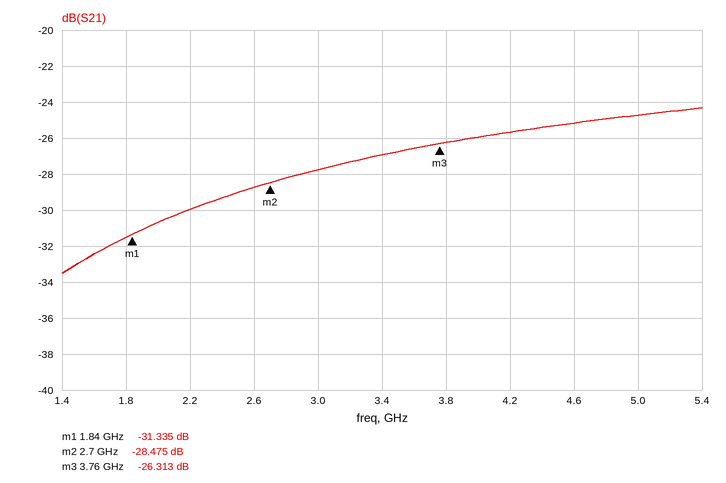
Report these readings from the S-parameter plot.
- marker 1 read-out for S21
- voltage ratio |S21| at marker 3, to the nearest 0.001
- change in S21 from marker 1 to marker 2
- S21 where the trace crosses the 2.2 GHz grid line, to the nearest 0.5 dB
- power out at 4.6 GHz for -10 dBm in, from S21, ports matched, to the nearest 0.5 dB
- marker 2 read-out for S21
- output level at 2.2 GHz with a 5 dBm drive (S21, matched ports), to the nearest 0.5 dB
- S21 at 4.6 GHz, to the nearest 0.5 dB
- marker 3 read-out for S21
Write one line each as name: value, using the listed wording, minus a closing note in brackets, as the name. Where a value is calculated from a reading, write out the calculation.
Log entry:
marker 1 read-out for S21: -31.335 dB
voltage ratio |S21| at marker 3, to the nearest 0.001: 10^(-26.313/20) ≈ 0.048
change in S21 from marker 1 to marker 2: -28.475 − (-31.335) = 2.860 dB
S21 where the trace crosses the 2.2 GHz grid line, to the nearest 0.5 dB: -30.0 dB
power out at 4.6 GHz for -10 dBm in, from S21, ports matched, to the nearest 0.5 dB: -10 dBm + (-25.0 dB) = -35.0 dBm
marker 2 read-out for S21: -28.475 dB
output level at 2.2 GHz with a 5 dBm drive (S21, matched ports), to the nearest 0.5 dB: 5 dBm + (-30.0 dB) = -25.0 dBm
S21 at 4.6 GHz, to the nearest 0.5 dB: -25.0 dB
marker 3 read-out for S21: -26.313 dB
